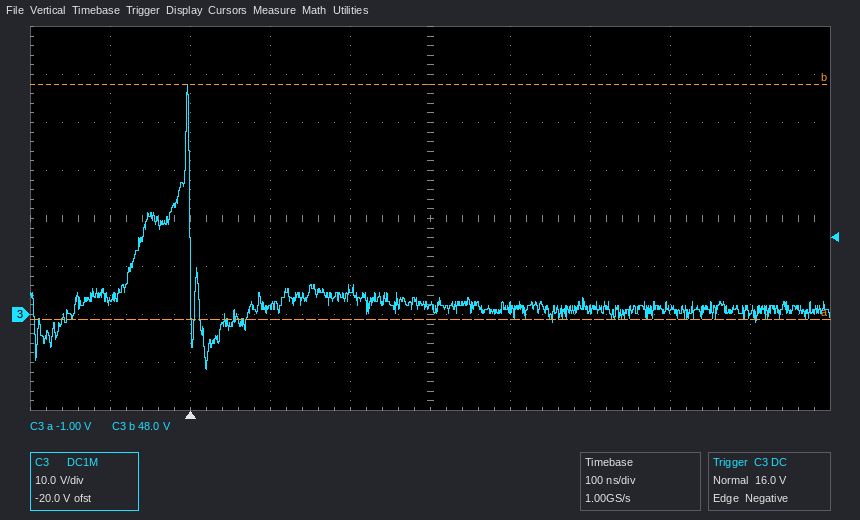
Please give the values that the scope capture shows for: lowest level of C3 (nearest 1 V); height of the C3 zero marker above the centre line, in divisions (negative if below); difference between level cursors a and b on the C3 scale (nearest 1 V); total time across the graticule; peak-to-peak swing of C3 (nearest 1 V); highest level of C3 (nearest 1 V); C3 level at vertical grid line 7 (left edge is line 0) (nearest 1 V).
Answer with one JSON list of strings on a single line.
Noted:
["-11 V", "-2.0 div", "49 V", "1 µs", "59 V", "48 V", "1 V"]
